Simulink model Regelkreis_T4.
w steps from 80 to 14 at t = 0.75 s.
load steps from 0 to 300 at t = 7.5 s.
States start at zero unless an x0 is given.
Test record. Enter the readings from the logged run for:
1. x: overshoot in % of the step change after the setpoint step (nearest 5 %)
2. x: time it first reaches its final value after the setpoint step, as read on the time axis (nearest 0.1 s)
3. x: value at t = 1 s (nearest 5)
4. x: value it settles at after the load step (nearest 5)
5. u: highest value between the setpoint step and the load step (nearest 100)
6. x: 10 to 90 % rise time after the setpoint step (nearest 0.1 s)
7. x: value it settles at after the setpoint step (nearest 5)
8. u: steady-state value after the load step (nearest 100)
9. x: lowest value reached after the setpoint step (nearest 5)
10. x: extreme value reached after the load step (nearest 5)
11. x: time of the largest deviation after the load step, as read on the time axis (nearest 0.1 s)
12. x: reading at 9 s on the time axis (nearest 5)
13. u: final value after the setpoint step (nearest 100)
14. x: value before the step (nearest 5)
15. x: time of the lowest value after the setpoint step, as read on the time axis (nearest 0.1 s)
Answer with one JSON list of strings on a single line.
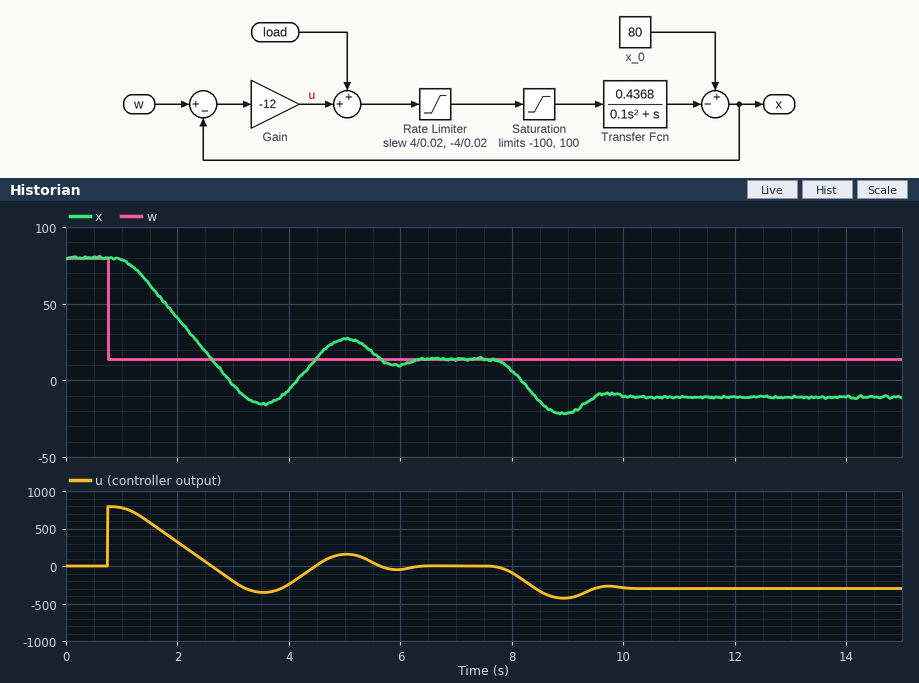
["45 %", "2.6 s", "80", "-10", "800", "1.2 s", "15", "-300", "-15", "-20", "8.9 s", "-20", "0", "80", "3.5 s"]
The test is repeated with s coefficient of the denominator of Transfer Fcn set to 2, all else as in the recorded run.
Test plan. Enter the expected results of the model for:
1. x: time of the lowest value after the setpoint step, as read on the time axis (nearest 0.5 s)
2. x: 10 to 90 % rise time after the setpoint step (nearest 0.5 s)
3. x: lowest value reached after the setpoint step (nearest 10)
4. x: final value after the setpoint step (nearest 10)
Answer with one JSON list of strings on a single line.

["4.5 s", "2.5 s", "10", "10"]
